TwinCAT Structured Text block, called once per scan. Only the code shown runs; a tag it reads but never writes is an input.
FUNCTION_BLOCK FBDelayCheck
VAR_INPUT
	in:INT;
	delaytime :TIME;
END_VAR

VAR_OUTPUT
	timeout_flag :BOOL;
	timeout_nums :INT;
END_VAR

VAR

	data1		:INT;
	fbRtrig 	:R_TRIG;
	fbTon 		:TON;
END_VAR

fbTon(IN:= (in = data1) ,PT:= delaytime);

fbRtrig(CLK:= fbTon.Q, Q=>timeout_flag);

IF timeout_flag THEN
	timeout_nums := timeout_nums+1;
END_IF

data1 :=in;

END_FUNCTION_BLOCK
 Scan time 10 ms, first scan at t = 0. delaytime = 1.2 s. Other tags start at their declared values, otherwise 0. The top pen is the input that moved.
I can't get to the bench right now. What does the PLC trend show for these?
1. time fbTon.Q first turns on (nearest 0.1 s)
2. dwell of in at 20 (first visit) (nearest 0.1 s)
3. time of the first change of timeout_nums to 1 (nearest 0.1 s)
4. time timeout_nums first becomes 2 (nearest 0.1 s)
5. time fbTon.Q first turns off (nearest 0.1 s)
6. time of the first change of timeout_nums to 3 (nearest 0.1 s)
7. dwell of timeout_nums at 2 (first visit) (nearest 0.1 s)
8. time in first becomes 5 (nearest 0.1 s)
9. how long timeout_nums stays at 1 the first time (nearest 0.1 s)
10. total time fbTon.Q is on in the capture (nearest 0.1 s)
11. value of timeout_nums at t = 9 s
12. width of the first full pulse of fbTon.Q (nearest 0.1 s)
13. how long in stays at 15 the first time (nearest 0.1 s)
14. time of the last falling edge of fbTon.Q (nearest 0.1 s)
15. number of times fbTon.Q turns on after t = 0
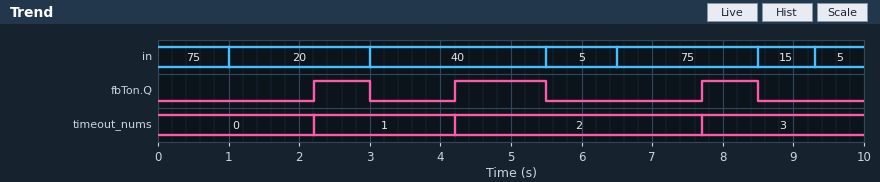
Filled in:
2.2 s
2.0 s
2.2 s
4.2 s
3.0 s
7.7 s
3.5 s
5.5 s
2.0 s
2.9 s
3
0.8 s
0.8 s
8.5 s
3
